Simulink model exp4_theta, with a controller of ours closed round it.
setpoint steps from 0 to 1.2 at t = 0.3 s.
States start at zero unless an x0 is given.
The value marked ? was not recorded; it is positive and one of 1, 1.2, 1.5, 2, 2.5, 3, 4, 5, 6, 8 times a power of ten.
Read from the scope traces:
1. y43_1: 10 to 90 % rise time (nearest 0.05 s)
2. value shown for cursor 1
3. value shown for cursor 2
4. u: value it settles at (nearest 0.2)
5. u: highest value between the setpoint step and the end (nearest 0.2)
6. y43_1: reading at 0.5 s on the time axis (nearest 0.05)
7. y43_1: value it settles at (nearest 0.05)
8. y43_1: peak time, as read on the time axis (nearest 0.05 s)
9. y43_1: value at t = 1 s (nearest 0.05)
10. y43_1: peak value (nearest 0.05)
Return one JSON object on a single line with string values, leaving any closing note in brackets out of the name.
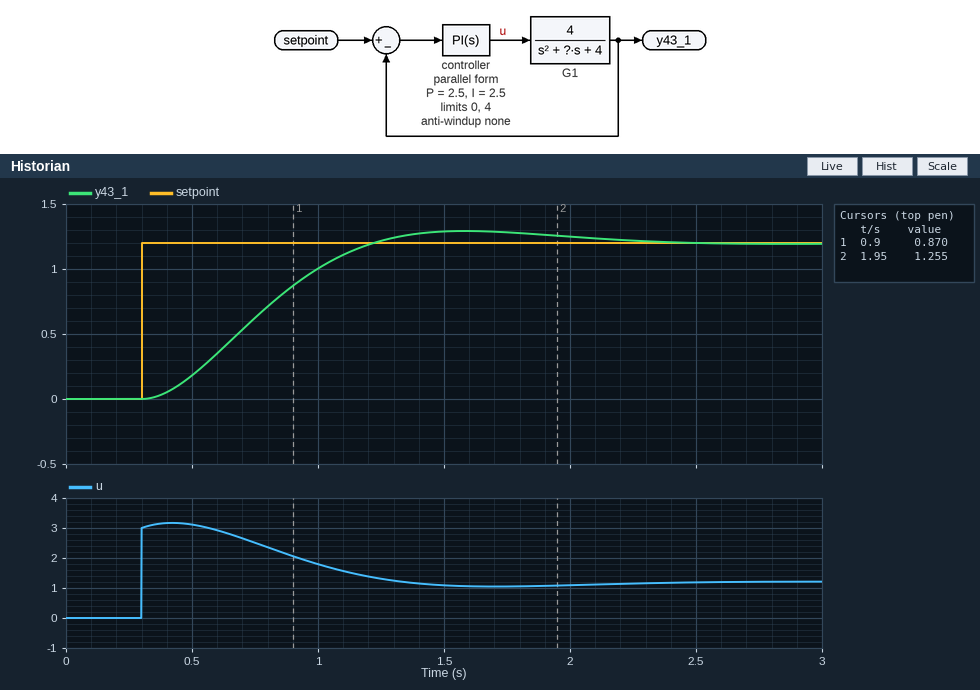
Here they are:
{"y43_1: 10 to 90 % rise time": "0.60 s", "value shown for cursor 1": "0.870", "value shown for cursor 2": "1.255", "u: value it settles at": "1.2", "u: highest value between the setpoint step and the end": "3.2", "y43_1: reading at 0.5 s on the time axis": "0.20", "y43_1: value it settles at": "1.20", "y43_1: peak time, as read on the time axis": "1.60 s", "y43_1: value at t = 1 s": "1.00", "y43_1: peak value": "1.30"}
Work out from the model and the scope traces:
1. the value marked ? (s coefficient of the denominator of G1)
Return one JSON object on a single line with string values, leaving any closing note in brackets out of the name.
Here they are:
{"the value marked ?": "5"}
